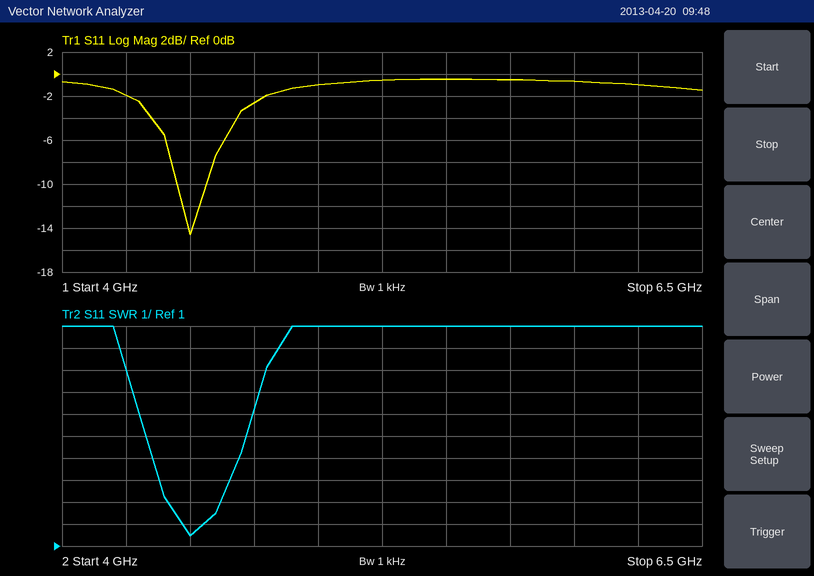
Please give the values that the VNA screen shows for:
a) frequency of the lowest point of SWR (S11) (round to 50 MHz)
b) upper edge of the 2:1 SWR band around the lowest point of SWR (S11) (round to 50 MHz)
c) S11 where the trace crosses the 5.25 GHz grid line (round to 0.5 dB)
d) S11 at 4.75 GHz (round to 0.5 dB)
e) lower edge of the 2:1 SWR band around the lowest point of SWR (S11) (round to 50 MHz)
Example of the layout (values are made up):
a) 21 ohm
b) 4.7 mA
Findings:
a) 4.50 GHz
b) 4.55 GHz
c) -0.5 dB
d) -2.5 dB
e) 4.45 GHz
